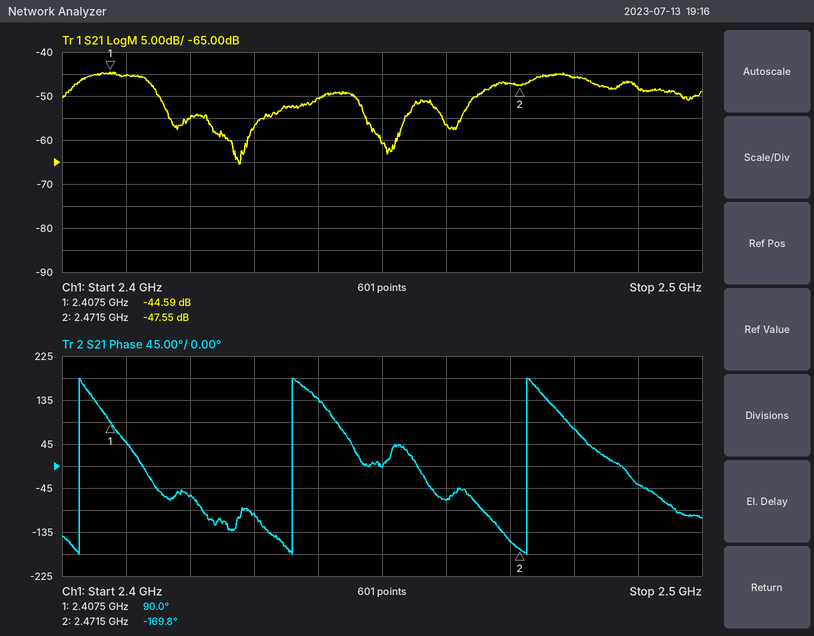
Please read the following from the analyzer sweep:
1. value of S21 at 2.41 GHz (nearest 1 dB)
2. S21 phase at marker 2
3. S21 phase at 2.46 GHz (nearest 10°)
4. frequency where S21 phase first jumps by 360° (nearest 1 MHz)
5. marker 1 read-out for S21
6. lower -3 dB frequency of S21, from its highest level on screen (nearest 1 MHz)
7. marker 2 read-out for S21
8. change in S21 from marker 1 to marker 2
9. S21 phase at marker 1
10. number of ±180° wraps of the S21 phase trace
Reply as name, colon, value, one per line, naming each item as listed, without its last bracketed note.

value of S21 at 2.41 GHz: -45 dB
S21 phase at marker 2: -169.8°
S21 phase at 2.46 GHz: -70°
frequency where S21 phase first jumps by 360°: 2.403 GHz
marker 1 read-out for S21: -44.59 dB
lower -3 dB frequency of S21, from its highest level on screen: 2.402 GHz
marker 2 read-out for S21: -47.55 dB
change in S21 from marker 1 to marker 2: -2.96 dB
S21 phase at marker 1: 90.0°
number of ±180° wraps of the S21 phase trace: 3
